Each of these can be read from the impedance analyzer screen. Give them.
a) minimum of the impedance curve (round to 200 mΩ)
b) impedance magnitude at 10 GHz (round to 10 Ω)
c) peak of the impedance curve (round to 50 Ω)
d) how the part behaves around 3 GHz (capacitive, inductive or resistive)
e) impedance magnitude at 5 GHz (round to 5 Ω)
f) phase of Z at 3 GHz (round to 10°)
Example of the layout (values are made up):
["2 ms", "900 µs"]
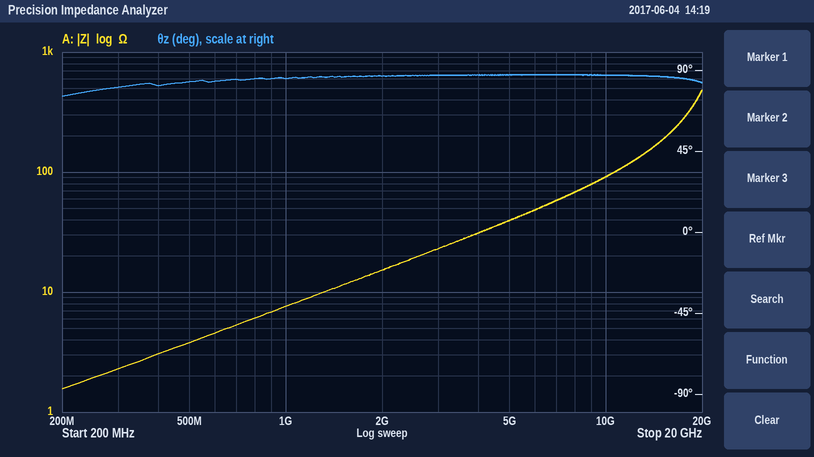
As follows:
["1.6 Ω", "90 Ω", "500 Ω", "inductive", "40 Ω", "90°"]
